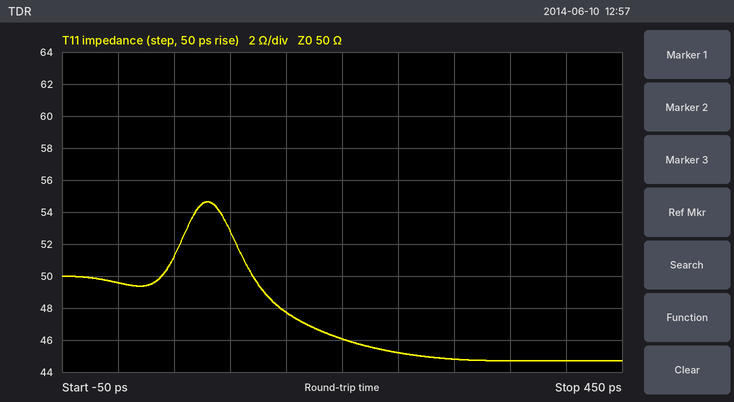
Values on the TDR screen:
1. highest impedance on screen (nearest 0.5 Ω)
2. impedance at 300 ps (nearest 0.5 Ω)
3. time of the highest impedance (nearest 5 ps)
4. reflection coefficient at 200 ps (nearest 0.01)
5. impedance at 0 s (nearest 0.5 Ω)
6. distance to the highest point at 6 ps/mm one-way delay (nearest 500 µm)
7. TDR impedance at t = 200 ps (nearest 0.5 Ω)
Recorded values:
54.5 Ω
45.0 Ω
80 ps
-0.04
49.5 Ω
6.5 mm
46.0 Ω
